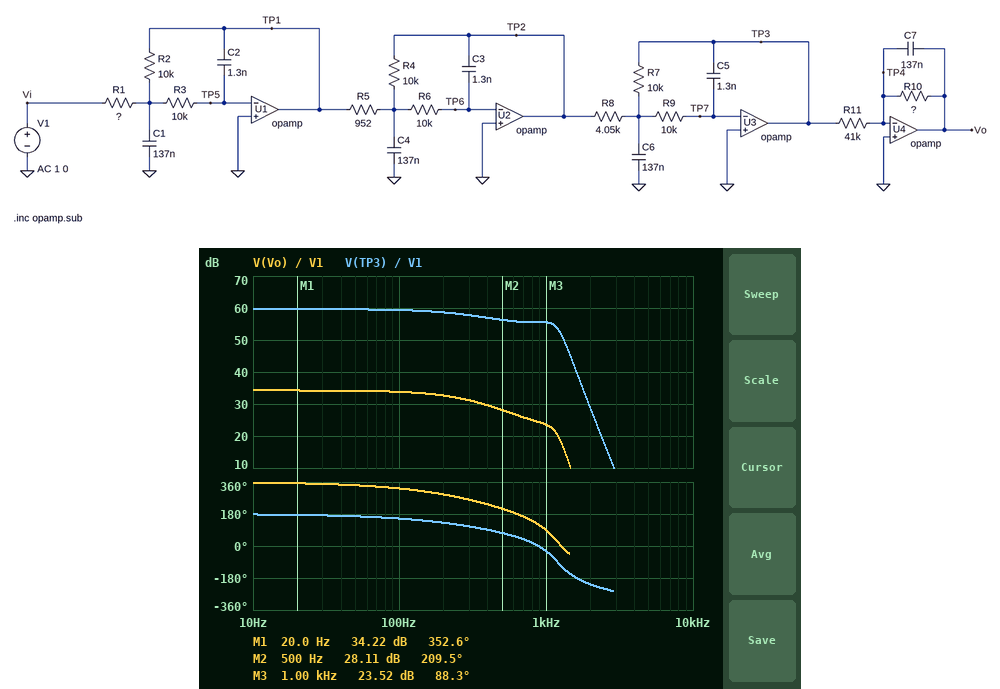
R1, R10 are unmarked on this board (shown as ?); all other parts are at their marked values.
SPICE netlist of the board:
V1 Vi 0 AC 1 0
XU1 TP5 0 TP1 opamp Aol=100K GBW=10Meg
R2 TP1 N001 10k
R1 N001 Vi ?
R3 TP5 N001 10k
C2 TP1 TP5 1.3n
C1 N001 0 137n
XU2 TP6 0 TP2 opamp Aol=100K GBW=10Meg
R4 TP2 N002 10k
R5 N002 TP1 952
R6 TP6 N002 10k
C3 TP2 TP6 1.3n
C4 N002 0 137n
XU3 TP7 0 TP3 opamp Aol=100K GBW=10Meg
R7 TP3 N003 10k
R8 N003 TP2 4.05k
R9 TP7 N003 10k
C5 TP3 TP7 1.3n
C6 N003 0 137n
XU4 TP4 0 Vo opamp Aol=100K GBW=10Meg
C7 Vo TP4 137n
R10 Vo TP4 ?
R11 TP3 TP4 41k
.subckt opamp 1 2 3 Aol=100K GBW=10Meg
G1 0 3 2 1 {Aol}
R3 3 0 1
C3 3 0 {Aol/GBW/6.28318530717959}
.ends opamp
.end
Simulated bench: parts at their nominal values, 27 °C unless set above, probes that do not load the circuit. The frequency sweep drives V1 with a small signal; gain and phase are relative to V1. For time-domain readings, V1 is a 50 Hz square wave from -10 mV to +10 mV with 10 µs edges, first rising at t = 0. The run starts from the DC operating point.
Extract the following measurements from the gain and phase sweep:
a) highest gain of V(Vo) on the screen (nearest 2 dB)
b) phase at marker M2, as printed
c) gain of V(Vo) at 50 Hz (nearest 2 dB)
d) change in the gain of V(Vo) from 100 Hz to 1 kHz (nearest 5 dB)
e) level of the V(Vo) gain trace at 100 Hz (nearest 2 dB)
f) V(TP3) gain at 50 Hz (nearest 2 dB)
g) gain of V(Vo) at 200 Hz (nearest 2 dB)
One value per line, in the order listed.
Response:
34 dB
209.5 deg
34 dB
-10 dB
34 dB
60 dB
32 dB
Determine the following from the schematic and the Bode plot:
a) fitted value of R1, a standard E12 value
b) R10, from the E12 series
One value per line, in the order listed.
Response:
270 Ω
2.2 kΩ
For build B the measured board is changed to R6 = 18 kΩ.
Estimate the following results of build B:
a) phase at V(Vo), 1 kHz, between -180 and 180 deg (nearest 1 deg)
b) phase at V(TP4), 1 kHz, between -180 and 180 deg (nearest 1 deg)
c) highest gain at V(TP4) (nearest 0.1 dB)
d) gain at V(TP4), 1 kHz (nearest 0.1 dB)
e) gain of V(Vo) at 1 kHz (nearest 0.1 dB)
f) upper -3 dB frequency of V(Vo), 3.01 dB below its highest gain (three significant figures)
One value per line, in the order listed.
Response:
64 deg
-32 deg
-58.9 dB
-61.0 dB
19.0 dB
272 Hz
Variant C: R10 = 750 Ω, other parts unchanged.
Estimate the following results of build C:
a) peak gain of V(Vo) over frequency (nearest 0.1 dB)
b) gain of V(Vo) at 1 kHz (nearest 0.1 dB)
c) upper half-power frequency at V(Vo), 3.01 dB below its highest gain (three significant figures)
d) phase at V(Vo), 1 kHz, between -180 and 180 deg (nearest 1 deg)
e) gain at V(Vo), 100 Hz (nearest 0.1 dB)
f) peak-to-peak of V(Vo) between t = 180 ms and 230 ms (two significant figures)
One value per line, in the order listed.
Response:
24.9 dB
19.3 dB
402 Hz
118 deg
24.6 dB
350 mV
